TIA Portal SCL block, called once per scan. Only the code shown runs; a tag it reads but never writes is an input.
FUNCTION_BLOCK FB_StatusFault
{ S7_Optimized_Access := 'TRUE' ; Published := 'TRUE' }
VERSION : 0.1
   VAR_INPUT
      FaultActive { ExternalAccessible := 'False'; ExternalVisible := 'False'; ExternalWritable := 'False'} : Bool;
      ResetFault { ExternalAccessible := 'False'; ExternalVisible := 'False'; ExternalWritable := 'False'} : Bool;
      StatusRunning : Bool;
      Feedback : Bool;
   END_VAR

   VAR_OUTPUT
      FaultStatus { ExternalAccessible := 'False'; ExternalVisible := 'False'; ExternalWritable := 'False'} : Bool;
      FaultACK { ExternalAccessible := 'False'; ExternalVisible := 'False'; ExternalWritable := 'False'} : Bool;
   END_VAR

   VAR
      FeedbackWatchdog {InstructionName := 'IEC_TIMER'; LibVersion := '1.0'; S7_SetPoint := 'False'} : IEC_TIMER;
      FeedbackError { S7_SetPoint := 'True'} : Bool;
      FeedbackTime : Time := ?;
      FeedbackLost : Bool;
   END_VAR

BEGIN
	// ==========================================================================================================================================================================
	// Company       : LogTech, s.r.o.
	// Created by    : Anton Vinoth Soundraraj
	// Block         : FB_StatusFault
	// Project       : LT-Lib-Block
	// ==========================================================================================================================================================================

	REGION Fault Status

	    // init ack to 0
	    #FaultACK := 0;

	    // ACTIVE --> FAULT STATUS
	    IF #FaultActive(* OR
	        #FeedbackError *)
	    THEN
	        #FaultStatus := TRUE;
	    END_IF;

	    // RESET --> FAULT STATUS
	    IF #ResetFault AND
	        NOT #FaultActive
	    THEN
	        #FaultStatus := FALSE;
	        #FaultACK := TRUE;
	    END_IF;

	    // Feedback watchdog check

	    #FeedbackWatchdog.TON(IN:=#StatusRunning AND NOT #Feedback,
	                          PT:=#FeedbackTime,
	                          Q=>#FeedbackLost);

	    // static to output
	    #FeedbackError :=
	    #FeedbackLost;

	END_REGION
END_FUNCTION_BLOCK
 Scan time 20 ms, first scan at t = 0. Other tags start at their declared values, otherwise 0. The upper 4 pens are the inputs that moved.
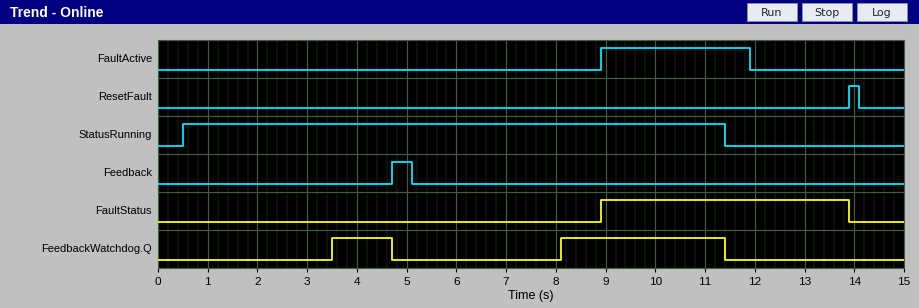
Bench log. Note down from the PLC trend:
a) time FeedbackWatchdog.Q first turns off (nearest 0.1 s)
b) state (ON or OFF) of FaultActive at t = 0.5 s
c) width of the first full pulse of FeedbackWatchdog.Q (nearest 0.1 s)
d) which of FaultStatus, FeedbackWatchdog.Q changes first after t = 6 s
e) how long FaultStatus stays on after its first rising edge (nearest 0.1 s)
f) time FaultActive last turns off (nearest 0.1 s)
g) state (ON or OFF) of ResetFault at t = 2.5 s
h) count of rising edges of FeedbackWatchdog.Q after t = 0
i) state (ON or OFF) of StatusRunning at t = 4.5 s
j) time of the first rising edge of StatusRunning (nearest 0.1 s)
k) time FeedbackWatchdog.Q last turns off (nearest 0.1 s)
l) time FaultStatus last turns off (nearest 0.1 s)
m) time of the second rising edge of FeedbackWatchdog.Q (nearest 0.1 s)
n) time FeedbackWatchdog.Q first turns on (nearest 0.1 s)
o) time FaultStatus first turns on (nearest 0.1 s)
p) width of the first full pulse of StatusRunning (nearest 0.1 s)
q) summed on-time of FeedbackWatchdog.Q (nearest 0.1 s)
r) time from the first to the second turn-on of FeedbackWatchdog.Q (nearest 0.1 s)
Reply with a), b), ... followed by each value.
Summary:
a) 4.7 s
b) OFF
c) 1.2 s
d) FeedbackWatchdog.Q
e) 5.0 s
f) 11.9 s
g) OFF
h) 2
i) ON
j) 0.5 s
k) 11.4 s
l) 13.9 s
m) 8.1 s
n) 3.5 s
o) 8.9 s
p) 10.9 s
q) 4.5 s
r) 4.6 s
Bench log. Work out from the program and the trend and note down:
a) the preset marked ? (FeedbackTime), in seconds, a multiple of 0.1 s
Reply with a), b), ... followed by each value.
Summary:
a) 3.0 s
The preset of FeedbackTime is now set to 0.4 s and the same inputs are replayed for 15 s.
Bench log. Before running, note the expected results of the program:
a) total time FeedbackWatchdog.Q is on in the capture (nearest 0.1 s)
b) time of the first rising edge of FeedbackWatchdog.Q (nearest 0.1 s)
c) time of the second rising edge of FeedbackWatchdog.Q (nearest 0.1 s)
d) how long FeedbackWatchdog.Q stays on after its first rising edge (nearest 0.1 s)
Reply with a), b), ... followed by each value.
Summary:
a) 9.7 s
b) 0.9 s
c) 5.5 s
d) 3.8 s
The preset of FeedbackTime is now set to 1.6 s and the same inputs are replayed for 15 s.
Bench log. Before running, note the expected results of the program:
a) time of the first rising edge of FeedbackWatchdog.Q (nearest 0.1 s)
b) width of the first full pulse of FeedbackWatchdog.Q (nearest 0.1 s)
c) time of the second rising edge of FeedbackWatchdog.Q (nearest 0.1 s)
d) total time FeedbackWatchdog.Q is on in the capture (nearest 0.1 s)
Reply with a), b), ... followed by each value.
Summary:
a) 2.1 s
b) 2.6 s
c) 6.7 s
d) 7.3 s
